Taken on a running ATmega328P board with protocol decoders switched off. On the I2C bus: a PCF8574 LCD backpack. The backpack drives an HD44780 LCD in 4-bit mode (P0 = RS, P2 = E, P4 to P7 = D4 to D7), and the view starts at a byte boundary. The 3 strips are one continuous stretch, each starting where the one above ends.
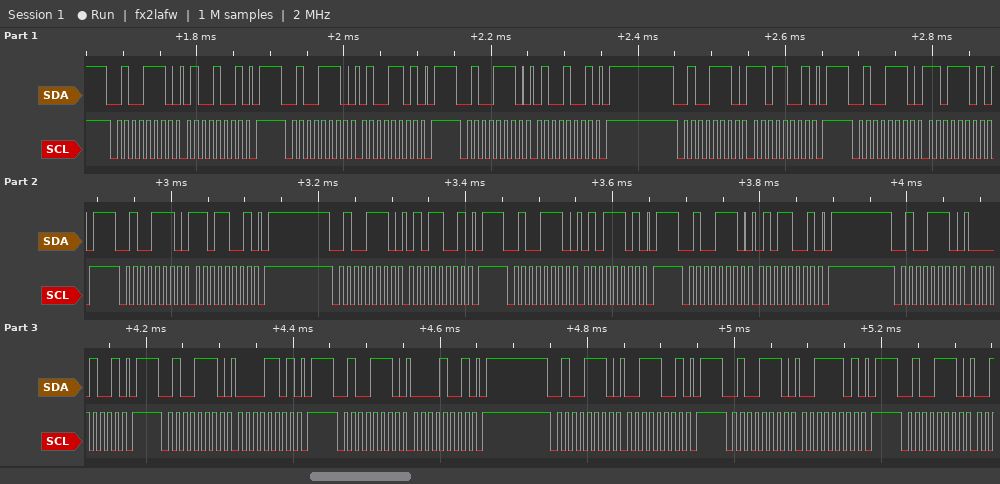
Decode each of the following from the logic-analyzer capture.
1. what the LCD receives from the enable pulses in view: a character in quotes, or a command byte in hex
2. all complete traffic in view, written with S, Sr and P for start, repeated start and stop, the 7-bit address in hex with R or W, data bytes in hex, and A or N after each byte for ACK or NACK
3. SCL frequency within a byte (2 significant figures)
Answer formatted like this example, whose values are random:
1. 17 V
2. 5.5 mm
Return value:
1. 'M' 'P'
2. S 27W A 49 A P S 27W A 4D A P S 27W A 49 A P S 27W A D9 A P S 27W A DD A P S 27W A D9 A P S 27W A 59 A P S 27W A 5D A P S 27W A 59 A P S 27W A 09 A P S 27W A 0D A P S 27W A 09 A P S 27W A 39 A P S 27W A 3D A P S 27W A
3. 100 kHz
